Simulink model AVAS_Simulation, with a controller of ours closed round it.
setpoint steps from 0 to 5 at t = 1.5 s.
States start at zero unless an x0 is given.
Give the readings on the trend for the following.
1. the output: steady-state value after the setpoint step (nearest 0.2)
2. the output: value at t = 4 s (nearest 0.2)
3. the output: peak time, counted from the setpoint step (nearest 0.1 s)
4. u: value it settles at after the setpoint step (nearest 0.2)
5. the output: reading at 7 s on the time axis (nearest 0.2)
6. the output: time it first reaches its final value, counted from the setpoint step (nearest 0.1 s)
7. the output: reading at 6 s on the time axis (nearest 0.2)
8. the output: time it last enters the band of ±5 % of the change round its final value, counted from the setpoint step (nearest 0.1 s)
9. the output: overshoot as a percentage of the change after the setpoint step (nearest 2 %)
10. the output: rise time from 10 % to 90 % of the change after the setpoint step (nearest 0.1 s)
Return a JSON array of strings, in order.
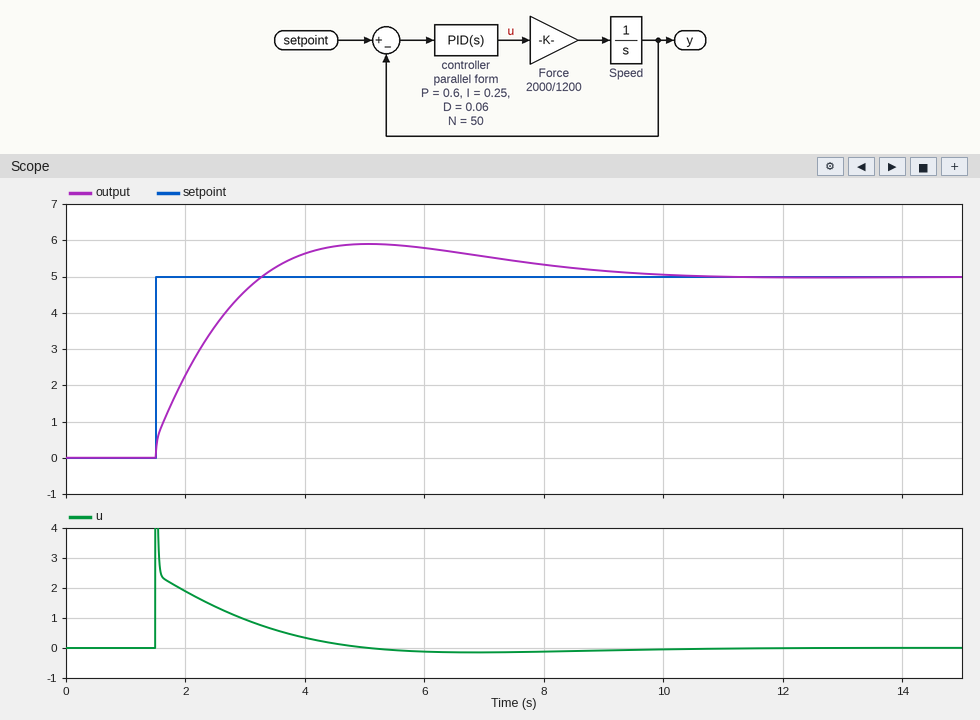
["5.0", "5.6", "3.6 s", "0.0", "5.6", "1.8 s", "5.8", "6.9 s", "18 %", "1.4 s"]
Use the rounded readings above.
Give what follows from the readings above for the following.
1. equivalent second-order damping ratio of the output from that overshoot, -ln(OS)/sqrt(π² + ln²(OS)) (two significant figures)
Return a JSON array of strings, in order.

["0.48"]
